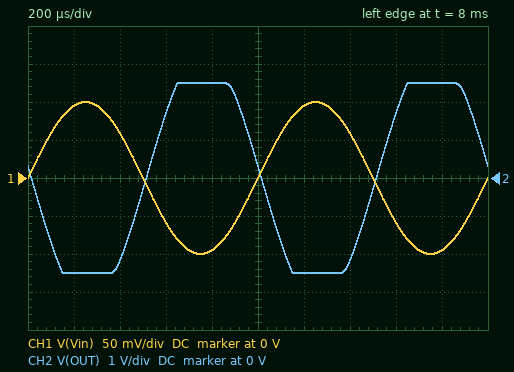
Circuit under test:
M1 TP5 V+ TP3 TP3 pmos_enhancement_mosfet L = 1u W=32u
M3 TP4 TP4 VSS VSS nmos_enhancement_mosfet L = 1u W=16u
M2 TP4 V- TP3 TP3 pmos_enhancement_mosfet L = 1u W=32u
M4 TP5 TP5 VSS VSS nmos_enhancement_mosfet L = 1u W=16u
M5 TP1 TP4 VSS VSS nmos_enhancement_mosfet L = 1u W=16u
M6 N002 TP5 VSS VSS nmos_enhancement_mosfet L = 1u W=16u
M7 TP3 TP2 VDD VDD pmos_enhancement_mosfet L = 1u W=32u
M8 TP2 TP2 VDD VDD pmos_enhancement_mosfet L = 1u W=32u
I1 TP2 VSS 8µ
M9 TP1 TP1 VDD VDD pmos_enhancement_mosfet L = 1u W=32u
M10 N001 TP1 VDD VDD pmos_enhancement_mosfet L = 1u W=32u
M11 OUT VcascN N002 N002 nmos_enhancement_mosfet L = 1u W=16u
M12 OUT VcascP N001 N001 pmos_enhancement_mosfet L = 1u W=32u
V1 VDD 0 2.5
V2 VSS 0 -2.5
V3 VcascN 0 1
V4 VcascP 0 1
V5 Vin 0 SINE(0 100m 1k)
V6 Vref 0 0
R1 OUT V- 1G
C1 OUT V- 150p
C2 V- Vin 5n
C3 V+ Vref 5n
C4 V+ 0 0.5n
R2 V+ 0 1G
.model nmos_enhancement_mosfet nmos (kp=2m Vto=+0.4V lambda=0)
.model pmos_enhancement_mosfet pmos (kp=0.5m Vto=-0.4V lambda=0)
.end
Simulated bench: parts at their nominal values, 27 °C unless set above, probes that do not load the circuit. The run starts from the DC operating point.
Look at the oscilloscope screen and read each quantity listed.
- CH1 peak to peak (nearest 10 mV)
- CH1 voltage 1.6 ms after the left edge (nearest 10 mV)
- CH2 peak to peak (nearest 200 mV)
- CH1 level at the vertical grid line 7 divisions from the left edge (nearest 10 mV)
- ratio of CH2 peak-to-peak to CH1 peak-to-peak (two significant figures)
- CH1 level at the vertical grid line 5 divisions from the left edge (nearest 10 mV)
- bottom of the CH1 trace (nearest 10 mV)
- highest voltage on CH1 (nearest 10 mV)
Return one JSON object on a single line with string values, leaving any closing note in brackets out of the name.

{"CH1 peak to peak": "200 mV", "CH1 voltage 1.6 ms after the left edge": "-60 mV", "CH2 peak to peak": "5.0 V", "CH1 level at the vertical grid line 7 divisions from the left edge": "60 mV", "ratio of CH2 peak-to-peak to CH1 peak-to-peak": "25", "CH1 level at the vertical grid line 5 divisions from the left edge": "0 V", "bottom of the CH1 trace": "-100 mV", "highest voltage on CH1": "100 mV"}
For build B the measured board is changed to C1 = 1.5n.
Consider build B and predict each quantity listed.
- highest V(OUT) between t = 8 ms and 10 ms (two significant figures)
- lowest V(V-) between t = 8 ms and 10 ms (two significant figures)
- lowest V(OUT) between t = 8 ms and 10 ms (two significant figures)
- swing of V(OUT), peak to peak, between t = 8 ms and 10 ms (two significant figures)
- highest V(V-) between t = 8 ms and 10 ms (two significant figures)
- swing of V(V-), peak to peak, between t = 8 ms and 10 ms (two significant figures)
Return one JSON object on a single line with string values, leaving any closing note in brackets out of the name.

{"highest V(OUT) between t = 8 ms and 10 ms": "330 mV", "lowest V(V-) between t = 8 ms and 10 ms": "-8.9 mV", "lowest V(OUT) between t = 8 ms and 10 ms": "-330 mV", "swing of V(OUT), peak to peak, between t = 8 ms and 10 ms": "660 mV", "highest V(V-) between t = 8 ms and 10 ms": "8.9 mV", "swing of V(V-), peak to peak, between t = 8 ms and 10 ms": "18 mV"}
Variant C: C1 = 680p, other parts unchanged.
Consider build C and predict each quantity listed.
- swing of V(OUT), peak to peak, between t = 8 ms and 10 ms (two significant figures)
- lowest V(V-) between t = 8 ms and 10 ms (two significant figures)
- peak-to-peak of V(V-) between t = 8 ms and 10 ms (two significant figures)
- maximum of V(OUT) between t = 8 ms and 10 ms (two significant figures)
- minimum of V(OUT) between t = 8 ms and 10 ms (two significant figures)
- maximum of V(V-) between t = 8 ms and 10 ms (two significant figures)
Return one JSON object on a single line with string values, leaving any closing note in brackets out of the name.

{"swing of V(OUT), peak to peak, between t = 8 ms and 10 ms": "1.5 V", "lowest V(V-) between t = 8 ms and 10 ms": "-8.9 mV", "peak-to-peak of V(V-) between t = 8 ms and 10 ms": "18 mV", "maximum of V(OUT) between t = 8 ms and 10 ms": "730 mV", "minimum of V(OUT) between t = 8 ms and 10 ms": "-730 mV", "maximum of V(V-) between t = 8 ms and 10 ms": "8.9 mV"}
